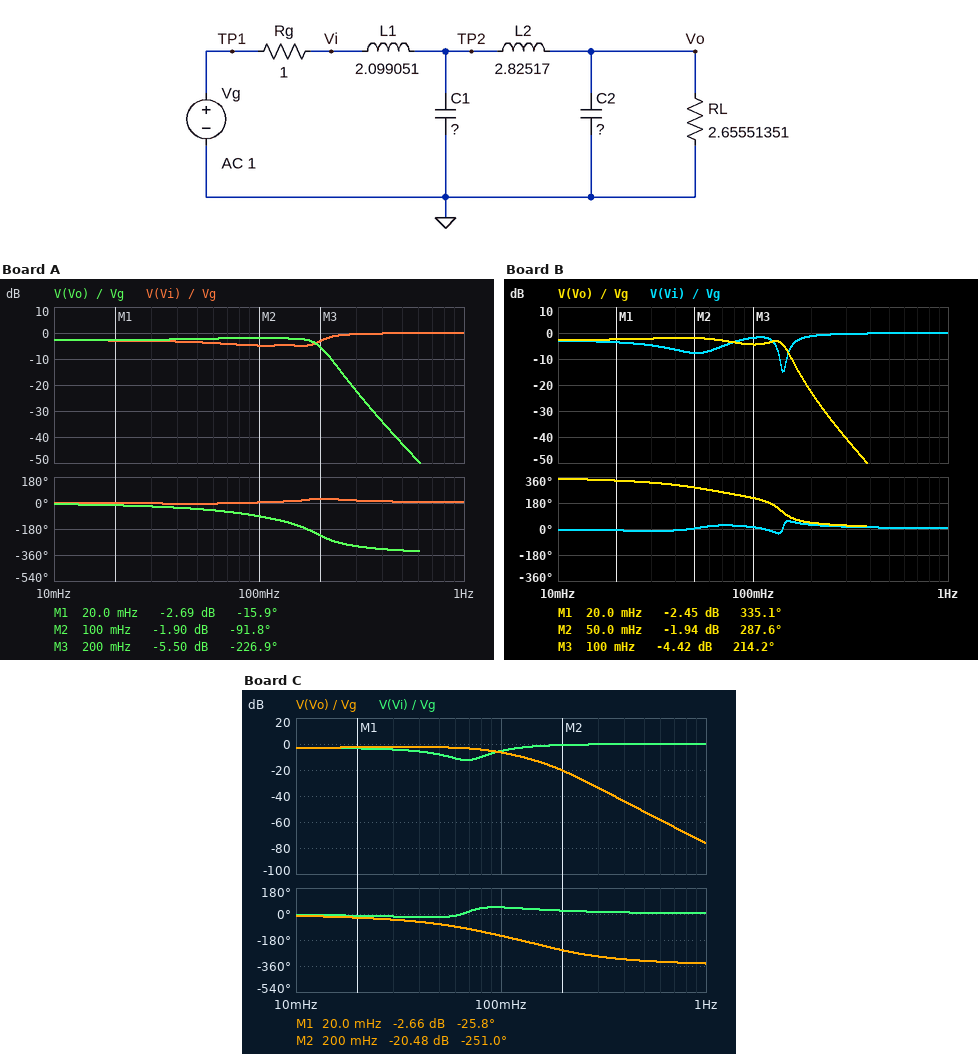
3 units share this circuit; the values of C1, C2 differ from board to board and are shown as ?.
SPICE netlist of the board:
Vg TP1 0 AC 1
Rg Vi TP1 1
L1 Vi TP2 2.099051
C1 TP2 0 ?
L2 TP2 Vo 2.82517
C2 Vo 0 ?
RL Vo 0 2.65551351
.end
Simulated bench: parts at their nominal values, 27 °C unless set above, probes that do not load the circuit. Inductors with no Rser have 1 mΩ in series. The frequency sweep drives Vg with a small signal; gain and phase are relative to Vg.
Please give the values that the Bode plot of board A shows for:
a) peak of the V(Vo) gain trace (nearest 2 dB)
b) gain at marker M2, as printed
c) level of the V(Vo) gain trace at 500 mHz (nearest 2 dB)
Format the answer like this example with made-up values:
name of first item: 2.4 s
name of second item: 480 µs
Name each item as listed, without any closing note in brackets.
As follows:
peak of the V(Vo) gain trace: -2 dB
gain at marker M2, as printed: -1.90 dB
level of the V(Vo) gain trace at 500 mHz: -42 dB
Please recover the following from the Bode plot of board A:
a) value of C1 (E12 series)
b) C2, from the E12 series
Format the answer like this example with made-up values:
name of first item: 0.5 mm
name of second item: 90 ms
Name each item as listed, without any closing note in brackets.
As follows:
value of C1: 820 mF
C2, from the E12 series: 330 mF
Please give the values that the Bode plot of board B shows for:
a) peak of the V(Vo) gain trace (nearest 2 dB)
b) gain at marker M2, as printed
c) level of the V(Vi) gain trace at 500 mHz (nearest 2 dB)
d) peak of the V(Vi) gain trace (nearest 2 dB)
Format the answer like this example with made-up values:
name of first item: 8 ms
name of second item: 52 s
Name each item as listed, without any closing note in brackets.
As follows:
peak of the V(Vo) gain trace: -2 dB
gain at marker M2, as printed: -1.94 dB
level of the V(Vi) gain trace at 500 mHz: 0 dB
peak of the V(Vi) gain trace: 0 dB
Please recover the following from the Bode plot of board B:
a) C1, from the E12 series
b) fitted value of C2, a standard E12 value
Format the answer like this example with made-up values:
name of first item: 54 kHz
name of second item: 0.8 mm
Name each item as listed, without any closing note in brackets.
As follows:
C1, from the E12 series: 1.2 F
fitted value of C2, a standard E12 value: 1.5 F
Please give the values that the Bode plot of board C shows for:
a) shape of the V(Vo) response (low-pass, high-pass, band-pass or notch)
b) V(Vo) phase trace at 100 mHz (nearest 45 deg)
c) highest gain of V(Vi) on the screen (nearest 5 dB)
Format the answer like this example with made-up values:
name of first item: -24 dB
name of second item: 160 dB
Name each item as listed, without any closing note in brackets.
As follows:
shape of the V(Vo) response: low-pass
V(Vo) phase trace at 100 mHz: -135 deg
highest gain of V(Vi) on the screen: 0 dB
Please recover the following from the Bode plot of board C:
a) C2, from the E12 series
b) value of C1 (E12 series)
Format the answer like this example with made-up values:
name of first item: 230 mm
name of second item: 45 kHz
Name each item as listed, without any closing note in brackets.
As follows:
C2, from the E12 series: 270 mF
value of C1: 2.7 F
